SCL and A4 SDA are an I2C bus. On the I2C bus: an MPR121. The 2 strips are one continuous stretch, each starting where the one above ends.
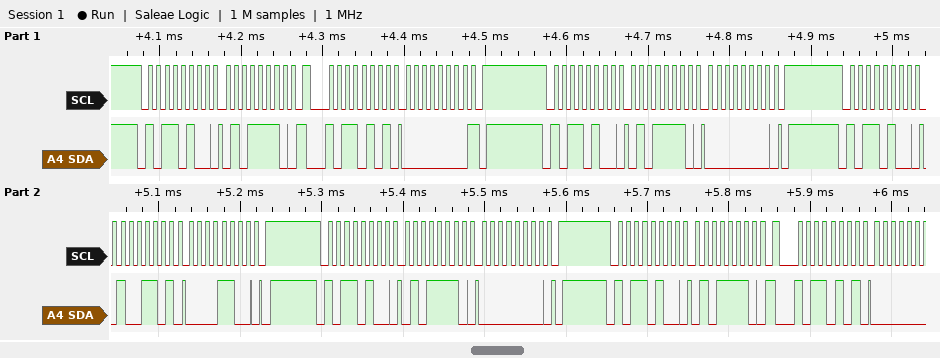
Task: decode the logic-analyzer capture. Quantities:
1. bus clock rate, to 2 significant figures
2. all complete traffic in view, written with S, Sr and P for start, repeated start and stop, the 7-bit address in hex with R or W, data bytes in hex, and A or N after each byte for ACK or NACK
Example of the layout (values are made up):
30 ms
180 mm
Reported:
100 kHz
S 5AW A 5E A Sr 5AR A 00 N P S 5AW A 5E A 00 A P S 5AW A 4D A 0C A P S 5AW A 5E A 00 A P S 5AW A 5E A Sr 5AR A
